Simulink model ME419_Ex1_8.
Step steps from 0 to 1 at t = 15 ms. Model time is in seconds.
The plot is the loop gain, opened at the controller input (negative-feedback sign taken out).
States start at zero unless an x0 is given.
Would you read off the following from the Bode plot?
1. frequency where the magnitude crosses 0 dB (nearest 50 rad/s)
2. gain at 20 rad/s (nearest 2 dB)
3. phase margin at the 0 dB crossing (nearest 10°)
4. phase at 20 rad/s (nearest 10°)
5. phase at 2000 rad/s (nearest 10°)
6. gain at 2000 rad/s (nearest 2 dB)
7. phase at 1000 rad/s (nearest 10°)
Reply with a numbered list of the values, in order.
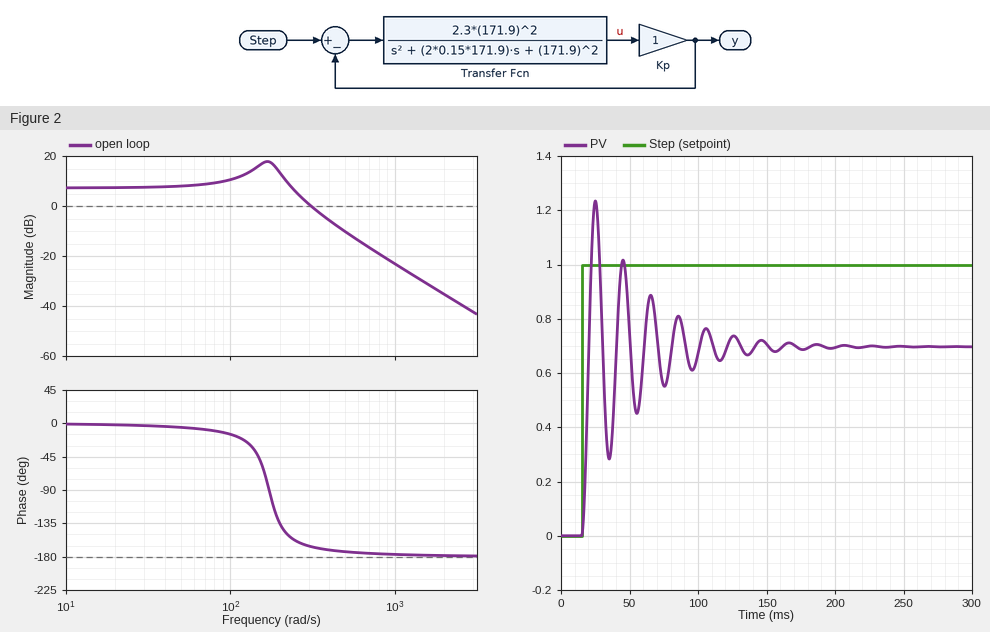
1. 300 rad/s
2. 8 dB
3. 10°
4. 0°
5. -180°
6. -36 dB
7. -180°
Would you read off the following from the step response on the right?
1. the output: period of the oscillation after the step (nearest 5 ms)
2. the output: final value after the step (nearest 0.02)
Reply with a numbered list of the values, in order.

1. 20 ms
2. 0.70
